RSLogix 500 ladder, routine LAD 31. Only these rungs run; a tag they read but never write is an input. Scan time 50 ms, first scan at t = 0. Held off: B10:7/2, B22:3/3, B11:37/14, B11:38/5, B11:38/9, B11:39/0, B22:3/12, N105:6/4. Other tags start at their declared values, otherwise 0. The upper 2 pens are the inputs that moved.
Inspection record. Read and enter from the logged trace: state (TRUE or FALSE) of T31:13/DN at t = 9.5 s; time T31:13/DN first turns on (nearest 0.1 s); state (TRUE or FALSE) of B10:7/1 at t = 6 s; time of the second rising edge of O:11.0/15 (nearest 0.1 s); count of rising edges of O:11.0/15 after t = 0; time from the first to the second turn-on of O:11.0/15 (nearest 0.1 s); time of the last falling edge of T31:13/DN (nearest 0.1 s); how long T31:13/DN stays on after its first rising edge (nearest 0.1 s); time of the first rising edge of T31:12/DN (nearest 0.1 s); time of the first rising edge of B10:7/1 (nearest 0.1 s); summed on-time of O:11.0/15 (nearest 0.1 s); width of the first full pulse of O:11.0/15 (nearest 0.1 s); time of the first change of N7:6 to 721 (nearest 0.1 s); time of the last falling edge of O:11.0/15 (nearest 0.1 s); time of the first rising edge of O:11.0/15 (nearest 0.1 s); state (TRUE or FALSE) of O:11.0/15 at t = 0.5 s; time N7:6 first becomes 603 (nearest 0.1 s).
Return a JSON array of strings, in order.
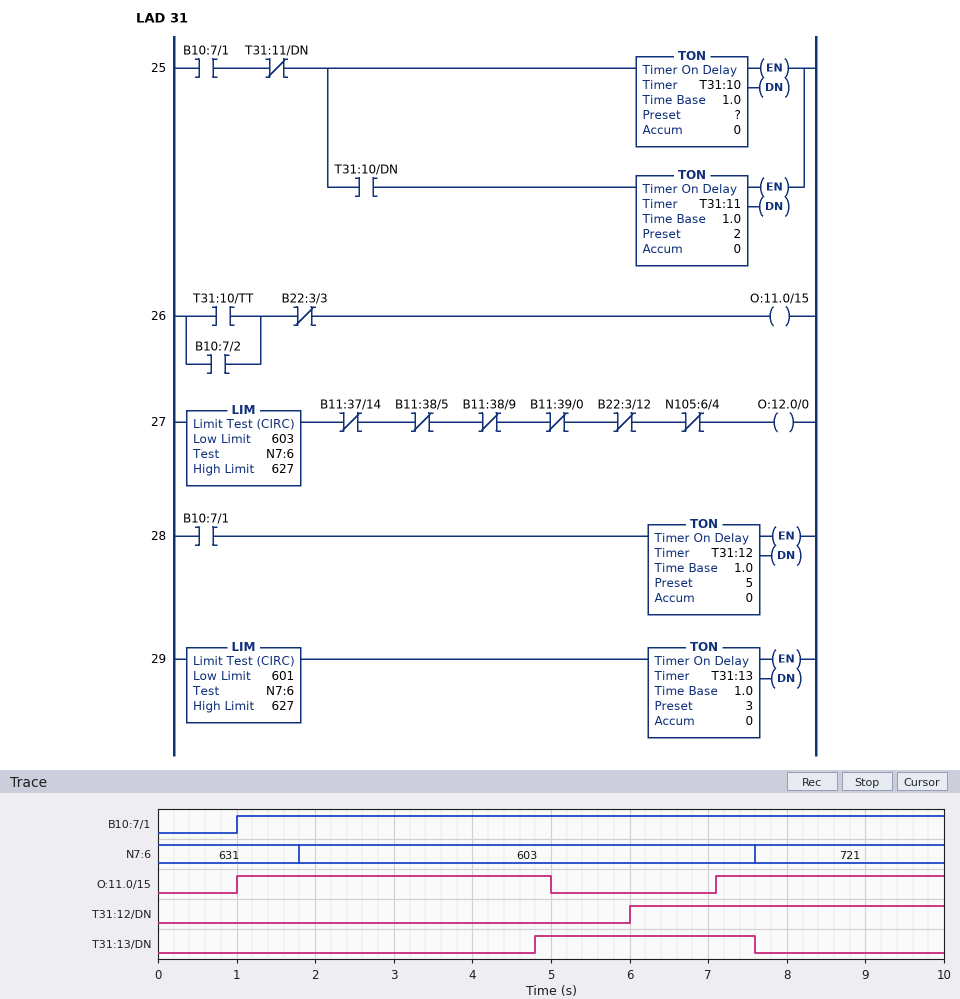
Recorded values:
["FALSE", "4.8 s", "TRUE", "7.1 s", "2", "6.1 s", "7.6 s", "2.8 s", "6.0 s", "1.0 s", "6.9 s", "4.0 s", "7.6 s", "5.0 s", "1.0 s", "FALSE", "1.8 s"]
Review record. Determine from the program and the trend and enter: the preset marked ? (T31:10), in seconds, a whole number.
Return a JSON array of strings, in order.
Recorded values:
["4 s"]
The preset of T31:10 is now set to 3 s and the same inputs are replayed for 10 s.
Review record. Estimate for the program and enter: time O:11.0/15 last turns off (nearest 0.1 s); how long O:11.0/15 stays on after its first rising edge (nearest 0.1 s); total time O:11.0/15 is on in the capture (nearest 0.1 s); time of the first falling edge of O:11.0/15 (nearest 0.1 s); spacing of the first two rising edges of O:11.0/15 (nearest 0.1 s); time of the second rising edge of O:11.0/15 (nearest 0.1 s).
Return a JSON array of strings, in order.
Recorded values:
["9.1 s", "3.0 s", "6.0 s", "4.0 s", "5.1 s", "6.1 s"]
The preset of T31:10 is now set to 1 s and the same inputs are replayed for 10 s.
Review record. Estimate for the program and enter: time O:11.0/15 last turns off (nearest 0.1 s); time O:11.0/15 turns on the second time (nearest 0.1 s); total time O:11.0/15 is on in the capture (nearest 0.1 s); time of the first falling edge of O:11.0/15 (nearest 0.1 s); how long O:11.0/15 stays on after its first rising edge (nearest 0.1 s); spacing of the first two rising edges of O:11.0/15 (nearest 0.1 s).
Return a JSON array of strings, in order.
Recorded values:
["8.2 s", "4.1 s", "3.0 s", "2.0 s", "1.0 s", "3.1 s"]
